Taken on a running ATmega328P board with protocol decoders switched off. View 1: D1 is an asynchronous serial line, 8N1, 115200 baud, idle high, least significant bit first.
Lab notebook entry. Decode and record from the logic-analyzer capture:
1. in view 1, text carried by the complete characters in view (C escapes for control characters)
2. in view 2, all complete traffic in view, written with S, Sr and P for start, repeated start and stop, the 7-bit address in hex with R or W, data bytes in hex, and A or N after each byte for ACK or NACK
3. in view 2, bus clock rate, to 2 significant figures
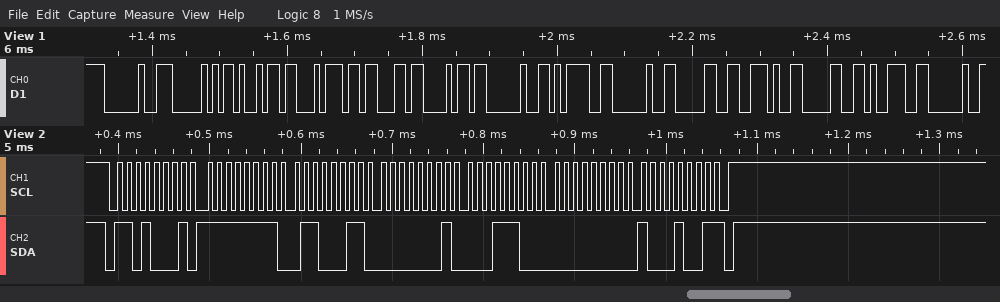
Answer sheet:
" Pitch = 0.09 "
S 68R A FF A 63 A 01 A 1C A 00 A 89 N P
100 kHz
